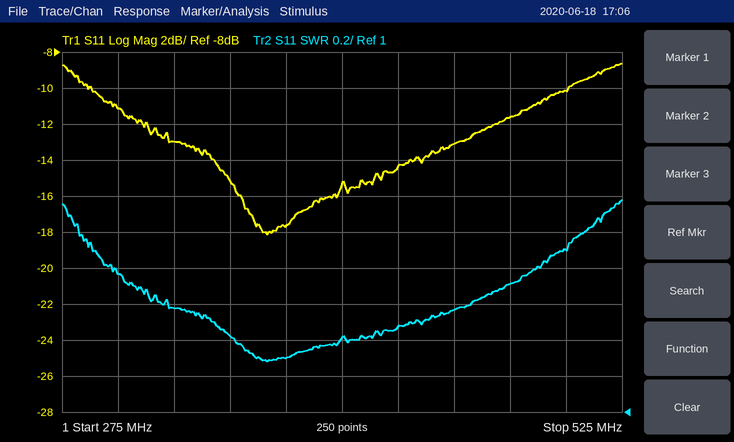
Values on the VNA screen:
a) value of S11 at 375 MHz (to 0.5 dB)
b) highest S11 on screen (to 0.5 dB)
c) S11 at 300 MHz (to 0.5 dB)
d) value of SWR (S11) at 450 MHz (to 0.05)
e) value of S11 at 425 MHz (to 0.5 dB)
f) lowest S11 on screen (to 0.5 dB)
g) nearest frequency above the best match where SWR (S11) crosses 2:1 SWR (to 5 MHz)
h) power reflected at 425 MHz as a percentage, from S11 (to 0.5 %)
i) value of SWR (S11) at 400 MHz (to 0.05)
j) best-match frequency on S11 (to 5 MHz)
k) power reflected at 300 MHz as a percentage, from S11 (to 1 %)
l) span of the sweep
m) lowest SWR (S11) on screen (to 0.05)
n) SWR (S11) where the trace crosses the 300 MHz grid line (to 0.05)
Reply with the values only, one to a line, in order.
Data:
-17.5 dB
-8.5 dB
-11.0 dB
1.55
-14.5 dB
-18.0 dB
510 MHz
3.5 %
1.40
365 MHz
8 %
250 MHz
1.30
1.75
